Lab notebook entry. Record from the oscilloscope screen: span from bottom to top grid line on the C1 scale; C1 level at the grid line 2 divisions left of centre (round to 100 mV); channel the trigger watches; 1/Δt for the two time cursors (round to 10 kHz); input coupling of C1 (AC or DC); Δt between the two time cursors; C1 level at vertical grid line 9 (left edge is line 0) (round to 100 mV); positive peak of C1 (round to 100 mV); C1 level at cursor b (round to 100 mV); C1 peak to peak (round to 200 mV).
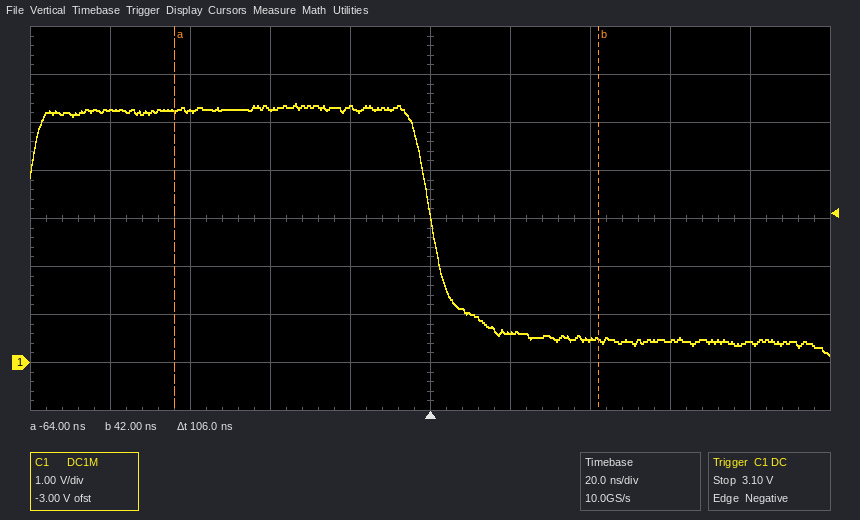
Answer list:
8 V
5.3 V
C1
9.43 MHz
DC
106 ns
400 mV
5.4 V
500 mV
5.2 V
